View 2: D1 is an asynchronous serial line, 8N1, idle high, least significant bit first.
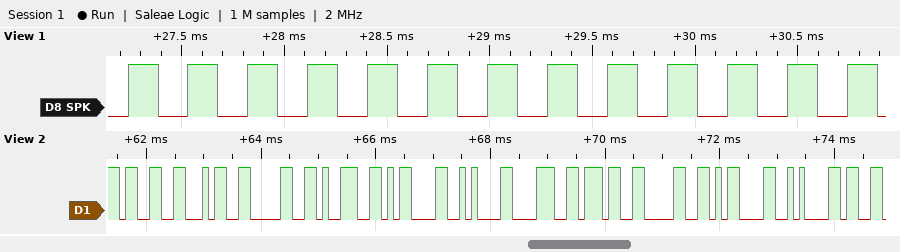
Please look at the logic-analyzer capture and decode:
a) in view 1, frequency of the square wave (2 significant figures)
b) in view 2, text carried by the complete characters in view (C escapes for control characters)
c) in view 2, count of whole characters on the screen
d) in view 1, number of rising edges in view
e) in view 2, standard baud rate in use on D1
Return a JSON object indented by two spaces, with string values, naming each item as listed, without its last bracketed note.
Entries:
{
  "in view 1, frequency of the square wave": "3.4 kHz",
  "in view 2, text carried by the complete characters in view": "\"3409\\r\\n870\\r\\n\"",
  "in view 2, count of whole characters on the screen": "11",
  "in view 1, number of rising edges in view": "13",
  "in view 2, standard baud rate in use on D1": "9600 baud"
}
